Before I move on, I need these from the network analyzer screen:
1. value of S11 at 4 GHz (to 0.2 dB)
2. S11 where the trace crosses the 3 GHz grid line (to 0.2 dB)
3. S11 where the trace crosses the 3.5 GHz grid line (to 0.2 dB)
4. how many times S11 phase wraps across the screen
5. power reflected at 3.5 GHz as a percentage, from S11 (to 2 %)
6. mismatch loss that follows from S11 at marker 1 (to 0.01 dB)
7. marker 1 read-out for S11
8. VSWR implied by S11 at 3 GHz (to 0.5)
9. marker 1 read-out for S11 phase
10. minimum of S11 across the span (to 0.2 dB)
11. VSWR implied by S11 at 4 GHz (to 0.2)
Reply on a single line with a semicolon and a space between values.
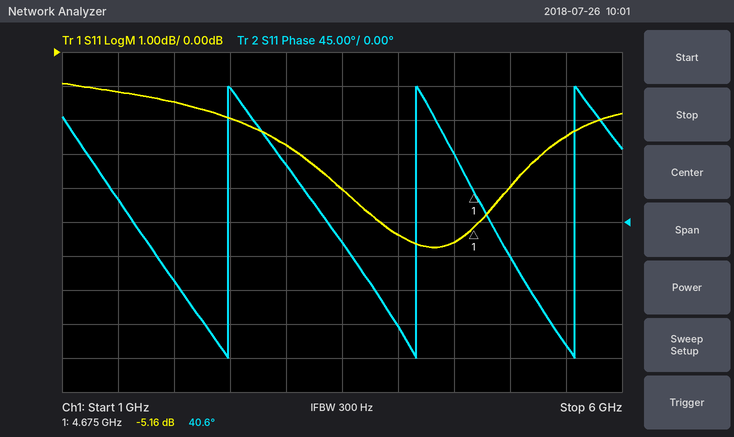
-5.4 dB; -2.8 dB; -4.0 dB; 3; 40 %; 1.58 dB; -5.16 dB; 6.5; 40.6°; -5.8 dB; 3.4
